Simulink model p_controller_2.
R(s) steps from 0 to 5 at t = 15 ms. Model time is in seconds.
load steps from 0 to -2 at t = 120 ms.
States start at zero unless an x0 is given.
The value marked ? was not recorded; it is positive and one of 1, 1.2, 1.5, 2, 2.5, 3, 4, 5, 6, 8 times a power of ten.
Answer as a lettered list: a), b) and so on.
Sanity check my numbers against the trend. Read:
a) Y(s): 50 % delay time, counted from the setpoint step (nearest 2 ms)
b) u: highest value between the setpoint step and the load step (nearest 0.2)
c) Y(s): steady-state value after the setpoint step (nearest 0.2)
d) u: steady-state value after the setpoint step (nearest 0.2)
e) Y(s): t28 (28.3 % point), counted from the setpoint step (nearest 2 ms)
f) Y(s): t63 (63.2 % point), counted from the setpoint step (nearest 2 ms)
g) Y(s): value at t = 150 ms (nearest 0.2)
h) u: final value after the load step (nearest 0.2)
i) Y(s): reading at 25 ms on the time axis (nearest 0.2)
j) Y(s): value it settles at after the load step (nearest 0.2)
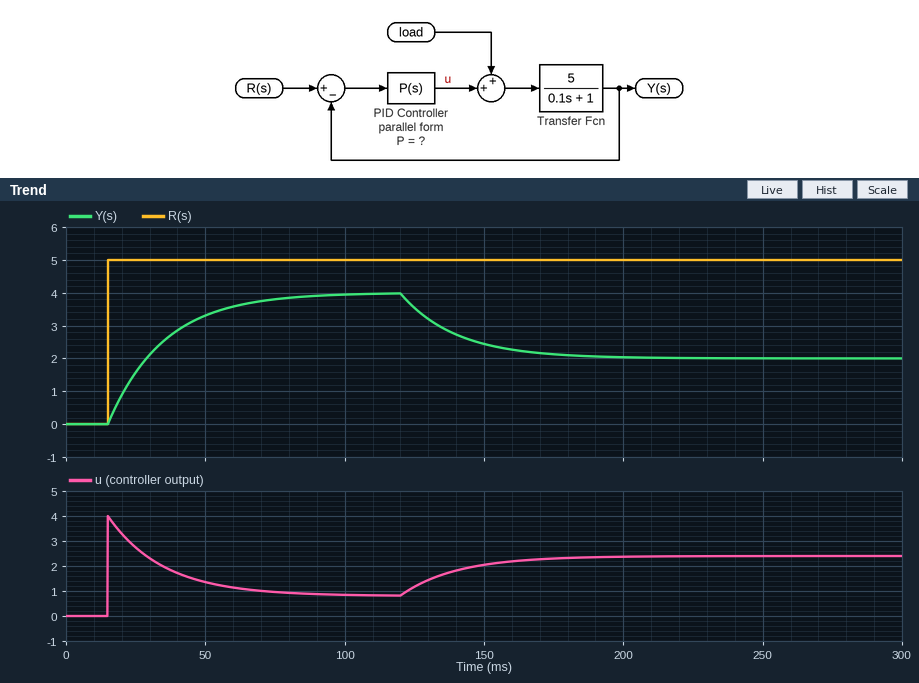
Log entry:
a) 14 ms
b) 4.0
c) 4.0
d) 0.8
e) 6 ms
f) 20 ms
g) 2.4
h) 2.4
i) 1.6
j) 2.0
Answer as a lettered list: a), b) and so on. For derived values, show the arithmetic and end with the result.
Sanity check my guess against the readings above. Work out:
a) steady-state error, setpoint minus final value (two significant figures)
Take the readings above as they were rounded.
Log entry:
a) 5 - 4 = 1.0
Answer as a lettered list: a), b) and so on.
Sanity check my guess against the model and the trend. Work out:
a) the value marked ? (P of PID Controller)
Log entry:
a) 0.8
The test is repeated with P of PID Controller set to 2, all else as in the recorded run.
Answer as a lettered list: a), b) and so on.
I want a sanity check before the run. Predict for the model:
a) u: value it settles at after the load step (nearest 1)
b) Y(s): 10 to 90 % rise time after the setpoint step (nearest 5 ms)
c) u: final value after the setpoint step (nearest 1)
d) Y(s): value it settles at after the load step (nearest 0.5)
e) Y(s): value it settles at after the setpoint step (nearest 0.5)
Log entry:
a) 3
b) 20 ms
c) 1
d) 3.5
e) 4.5
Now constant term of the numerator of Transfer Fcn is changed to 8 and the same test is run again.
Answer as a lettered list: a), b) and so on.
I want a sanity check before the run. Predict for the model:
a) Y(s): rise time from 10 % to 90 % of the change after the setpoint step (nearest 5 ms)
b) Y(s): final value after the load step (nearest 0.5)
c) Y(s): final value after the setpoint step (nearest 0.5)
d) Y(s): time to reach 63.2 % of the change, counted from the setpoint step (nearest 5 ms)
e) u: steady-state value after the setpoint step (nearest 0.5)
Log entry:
a) 30 ms
b) 2.0
c) 4.5
d) 15 ms
e) 0.5
